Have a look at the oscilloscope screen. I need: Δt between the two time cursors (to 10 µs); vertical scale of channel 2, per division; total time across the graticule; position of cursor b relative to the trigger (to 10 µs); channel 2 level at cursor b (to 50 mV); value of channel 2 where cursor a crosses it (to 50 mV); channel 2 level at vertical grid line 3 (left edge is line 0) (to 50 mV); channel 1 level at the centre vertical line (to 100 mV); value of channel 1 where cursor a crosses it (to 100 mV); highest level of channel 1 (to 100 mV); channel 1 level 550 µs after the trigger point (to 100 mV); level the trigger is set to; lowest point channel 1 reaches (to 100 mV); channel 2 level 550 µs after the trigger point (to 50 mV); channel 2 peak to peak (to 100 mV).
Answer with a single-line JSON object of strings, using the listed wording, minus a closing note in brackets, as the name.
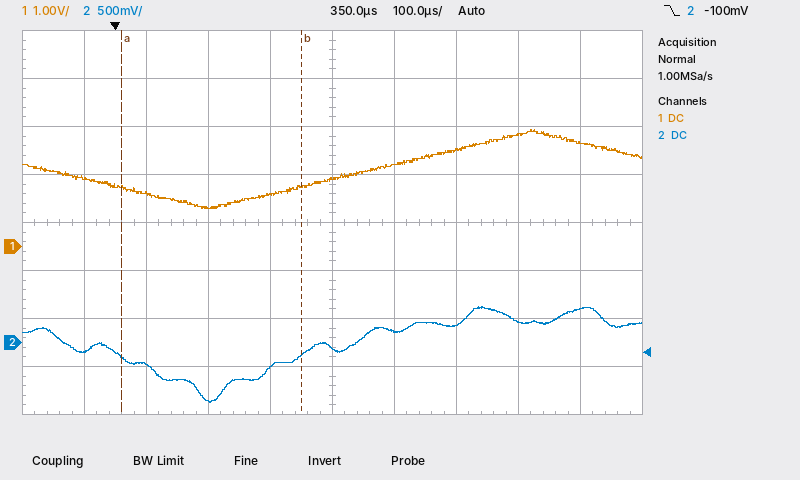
{"Δt between the two time cursors": "290 µs", "vertical scale of channel 2, per division": "500 mV", "total time across the graticule": "1 ms", "position of cursor b relative to the trigger": "+300 µs", "channel 2 level at cursor b": "-150 mV", "value of channel 2 where cursor a crosses it": "-150 mV", "channel 2 level at vertical grid line 3 (left edge is line 0)": "-600 mV", "channel 1 level at the centre vertical line": "1.4 V", "value of channel 1 where cursor a crosses it": "1.2 V", "highest level of channel 1": "2.4 V", "channel 1 level 550 µs after the trigger point": "2.0 V", "level the trigger is set to": "-100 mV", "lowest point channel 1 reaches": "800 mV", "channel 2 level 550 µs after the trigger point": "200 mV", "channel 2 peak to peak": "1.00 V"}
